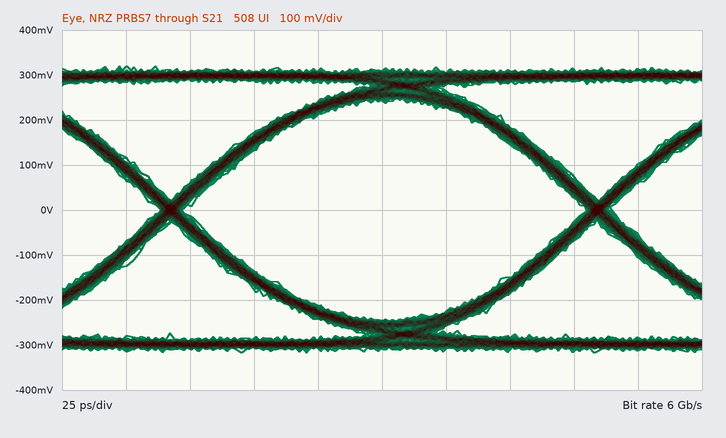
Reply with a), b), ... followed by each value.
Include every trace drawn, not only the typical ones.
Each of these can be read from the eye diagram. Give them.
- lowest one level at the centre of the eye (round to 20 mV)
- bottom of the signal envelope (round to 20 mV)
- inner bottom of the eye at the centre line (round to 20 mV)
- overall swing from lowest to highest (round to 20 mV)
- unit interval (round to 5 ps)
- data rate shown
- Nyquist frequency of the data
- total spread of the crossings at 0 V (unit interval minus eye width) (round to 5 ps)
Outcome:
a) 240 mV
b) -320 mV
c) -240 mV
d) 640 mV
e) 165 ps
f) 6 Gb/s
g) 3 GHz
h) 10 ps
